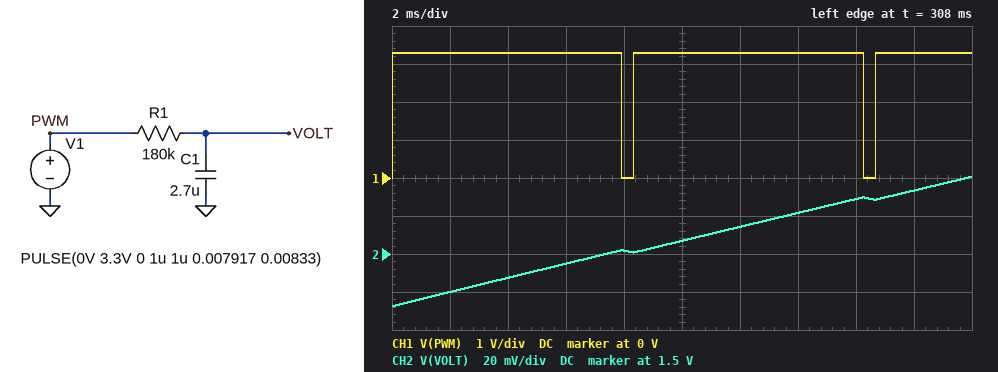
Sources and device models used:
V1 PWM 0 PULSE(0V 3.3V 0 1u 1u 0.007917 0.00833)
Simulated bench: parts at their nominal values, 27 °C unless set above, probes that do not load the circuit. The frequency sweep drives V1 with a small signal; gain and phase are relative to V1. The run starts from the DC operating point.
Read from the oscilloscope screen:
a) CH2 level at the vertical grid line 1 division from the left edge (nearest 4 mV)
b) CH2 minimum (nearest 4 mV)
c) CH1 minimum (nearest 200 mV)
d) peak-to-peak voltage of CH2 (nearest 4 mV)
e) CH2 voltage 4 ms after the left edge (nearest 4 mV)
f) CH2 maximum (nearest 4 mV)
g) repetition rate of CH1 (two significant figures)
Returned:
1.480 V
1.472 V
0 V
68 mV
1.488 V
1.540 V
120 Hz
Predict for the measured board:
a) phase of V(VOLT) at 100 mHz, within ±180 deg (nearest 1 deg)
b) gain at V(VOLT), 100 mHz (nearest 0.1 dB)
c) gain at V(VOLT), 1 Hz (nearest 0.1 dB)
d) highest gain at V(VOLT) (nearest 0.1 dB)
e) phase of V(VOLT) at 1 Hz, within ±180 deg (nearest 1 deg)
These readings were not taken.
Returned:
-17 deg
-0.4 dB
-10.1 dB
0 dB
-72 deg
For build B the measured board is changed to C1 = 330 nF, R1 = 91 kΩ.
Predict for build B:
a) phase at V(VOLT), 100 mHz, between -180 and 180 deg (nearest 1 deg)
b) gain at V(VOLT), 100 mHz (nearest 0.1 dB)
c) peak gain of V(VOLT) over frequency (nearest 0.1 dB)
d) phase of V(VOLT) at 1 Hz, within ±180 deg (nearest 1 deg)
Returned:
-1 deg
0 dB
0 dB
-11 deg
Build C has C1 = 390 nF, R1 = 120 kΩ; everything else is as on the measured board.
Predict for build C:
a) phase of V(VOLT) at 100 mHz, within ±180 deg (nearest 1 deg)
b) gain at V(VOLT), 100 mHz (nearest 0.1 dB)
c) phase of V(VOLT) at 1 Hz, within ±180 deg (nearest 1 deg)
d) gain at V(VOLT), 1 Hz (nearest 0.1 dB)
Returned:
-2 deg
0 dB
-16 deg
-0.4 dB
